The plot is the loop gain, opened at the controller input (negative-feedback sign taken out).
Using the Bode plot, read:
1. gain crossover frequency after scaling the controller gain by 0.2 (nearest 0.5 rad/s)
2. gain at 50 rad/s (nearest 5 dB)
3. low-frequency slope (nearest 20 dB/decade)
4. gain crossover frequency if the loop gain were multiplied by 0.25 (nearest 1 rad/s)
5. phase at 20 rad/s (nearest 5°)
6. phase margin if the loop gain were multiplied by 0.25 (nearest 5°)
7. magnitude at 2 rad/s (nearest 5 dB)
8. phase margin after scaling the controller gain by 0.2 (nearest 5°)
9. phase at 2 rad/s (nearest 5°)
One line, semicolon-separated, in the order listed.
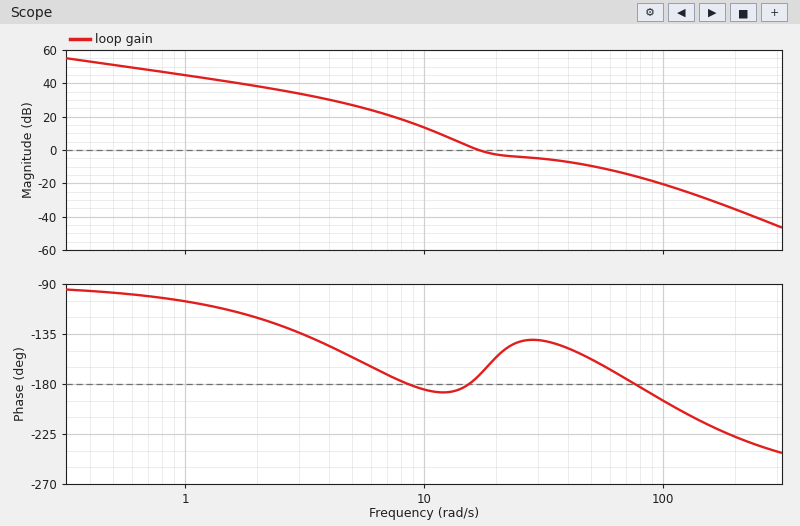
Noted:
10.0 rad/s; -10 dB; -20 dB/decade; 11 rad/s; -155°; -5°; 40 dB; -5°; -120°
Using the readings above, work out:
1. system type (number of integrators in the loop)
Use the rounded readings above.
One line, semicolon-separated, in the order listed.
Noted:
1
